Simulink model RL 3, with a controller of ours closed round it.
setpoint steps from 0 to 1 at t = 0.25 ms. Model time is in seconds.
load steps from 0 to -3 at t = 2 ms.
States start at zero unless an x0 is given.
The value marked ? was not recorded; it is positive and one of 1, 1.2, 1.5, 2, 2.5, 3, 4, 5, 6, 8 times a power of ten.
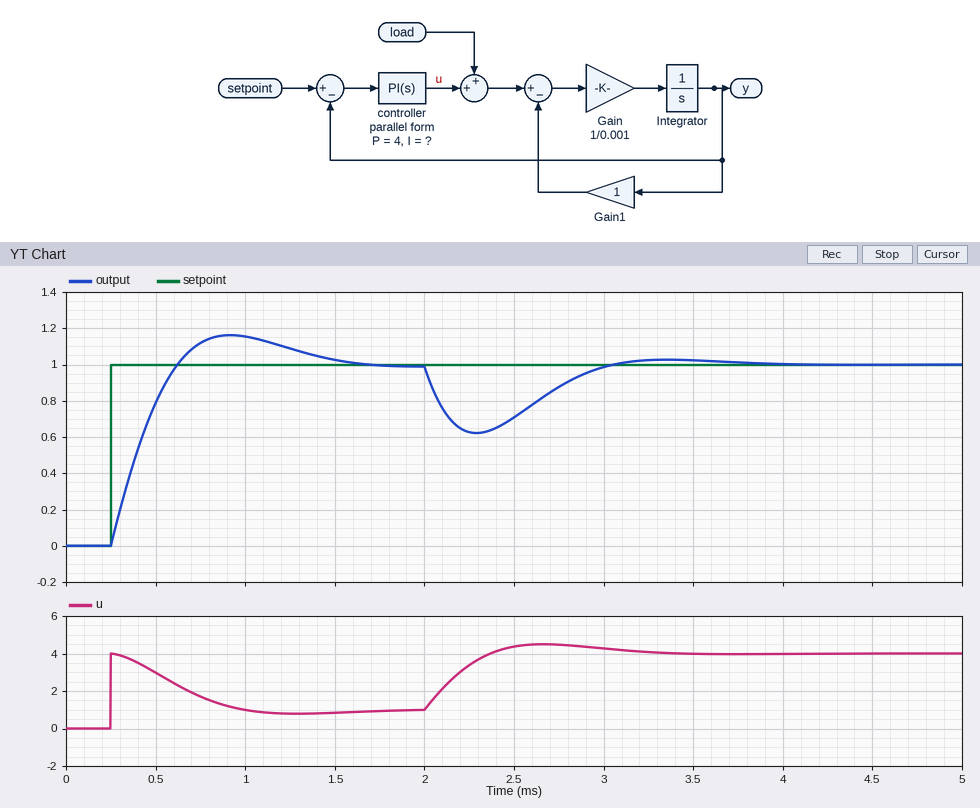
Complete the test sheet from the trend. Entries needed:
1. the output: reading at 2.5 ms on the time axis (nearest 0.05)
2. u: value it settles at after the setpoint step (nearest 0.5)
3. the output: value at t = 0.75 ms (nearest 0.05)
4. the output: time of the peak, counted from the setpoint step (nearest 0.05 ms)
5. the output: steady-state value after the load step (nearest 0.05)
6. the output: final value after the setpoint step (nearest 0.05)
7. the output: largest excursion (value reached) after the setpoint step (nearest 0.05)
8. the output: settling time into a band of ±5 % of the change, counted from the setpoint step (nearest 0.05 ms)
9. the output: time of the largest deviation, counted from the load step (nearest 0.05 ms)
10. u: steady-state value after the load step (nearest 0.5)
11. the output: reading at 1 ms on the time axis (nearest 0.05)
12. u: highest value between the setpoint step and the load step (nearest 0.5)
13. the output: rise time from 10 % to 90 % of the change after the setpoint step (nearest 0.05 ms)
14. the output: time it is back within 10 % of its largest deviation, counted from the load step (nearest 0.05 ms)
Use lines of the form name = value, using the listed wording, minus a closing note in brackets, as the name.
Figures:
the output: reading at 2.5 ms on the time axis = 0.70
u: value it settles at after the setpoint step = 1.0
the output: value at t = 0.75 ms = 1.10
the output: time of the peak, counted from the setpoint step = 0.65 ms
the output: steady-state value after the load step = 1.00
the output: final value after the setpoint step = 1.00
the output: largest excursion (value reached) after the setpoint step = 1.15
the output: settling time into a band of ±5 % of the change, counted from the setpoint step = 1.15 ms
the output: time of the largest deviation, counted from the load step = 0.30 ms
u: steady-state value after the load step = 4.0
the output: reading at 1 ms on the time axis = 1.15
u: highest value between the setpoint step and the load step = 4.0
the output: rise time from 10 % to 90 % of the change after the setpoint step = 0.30 ms
the output: time it is back within 10 % of its largest deviation, counted from the load step = 0.95 ms
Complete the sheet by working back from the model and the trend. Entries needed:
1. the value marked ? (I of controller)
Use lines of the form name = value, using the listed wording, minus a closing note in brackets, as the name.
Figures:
the value marked ? = 15000
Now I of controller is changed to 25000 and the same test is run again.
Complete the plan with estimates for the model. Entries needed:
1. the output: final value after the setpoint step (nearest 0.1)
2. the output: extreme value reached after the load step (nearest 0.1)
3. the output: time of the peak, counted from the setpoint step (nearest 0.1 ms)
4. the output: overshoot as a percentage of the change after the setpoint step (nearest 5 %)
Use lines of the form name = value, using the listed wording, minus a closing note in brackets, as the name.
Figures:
the output: final value after the setpoint step = 1.0
the output: extreme value reached after the load step = 0.7
the output: time of the peak, counted from the setpoint step = 0.5 ms
the output: overshoot as a percentage of the change after the setpoint step = 25 %
